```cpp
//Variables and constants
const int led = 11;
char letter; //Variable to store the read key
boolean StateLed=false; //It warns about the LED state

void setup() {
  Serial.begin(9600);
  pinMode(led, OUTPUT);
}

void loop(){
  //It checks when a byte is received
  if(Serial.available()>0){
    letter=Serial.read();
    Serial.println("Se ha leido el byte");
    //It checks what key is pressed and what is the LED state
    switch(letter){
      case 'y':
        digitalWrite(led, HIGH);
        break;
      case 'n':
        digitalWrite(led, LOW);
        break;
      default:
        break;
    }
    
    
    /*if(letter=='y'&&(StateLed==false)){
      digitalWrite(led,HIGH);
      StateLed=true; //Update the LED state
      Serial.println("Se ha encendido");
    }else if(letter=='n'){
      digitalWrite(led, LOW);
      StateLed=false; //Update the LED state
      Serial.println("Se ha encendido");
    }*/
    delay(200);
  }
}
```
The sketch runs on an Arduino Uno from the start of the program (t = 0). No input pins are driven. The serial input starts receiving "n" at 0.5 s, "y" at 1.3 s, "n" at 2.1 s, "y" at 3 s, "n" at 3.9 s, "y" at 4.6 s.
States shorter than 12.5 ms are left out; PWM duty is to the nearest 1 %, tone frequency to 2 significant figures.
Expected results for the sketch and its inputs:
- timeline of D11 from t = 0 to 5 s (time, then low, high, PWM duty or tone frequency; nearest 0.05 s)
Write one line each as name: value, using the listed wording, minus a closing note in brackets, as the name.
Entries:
timeline of D11 from t = 0 to 5 s: 0 s low; 1.3 s high; 2.1 s low; 3 s high; 3.9 s low; 4.6 s high
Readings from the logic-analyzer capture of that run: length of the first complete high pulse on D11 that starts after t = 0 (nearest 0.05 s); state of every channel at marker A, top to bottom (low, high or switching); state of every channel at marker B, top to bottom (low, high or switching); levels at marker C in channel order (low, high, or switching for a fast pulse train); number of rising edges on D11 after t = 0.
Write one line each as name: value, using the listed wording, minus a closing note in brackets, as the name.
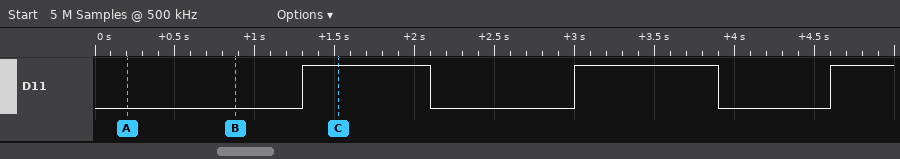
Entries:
length of the first complete high pulse on D11 that starts after t = 0: 0.80 s
state of every channel at marker A, top to bottom: D11 low
state of every channel at marker B, top to bottom: D11 low
levels at marker C in channel order: D11 high
number of rising edges on D11 after t = 0: 3
